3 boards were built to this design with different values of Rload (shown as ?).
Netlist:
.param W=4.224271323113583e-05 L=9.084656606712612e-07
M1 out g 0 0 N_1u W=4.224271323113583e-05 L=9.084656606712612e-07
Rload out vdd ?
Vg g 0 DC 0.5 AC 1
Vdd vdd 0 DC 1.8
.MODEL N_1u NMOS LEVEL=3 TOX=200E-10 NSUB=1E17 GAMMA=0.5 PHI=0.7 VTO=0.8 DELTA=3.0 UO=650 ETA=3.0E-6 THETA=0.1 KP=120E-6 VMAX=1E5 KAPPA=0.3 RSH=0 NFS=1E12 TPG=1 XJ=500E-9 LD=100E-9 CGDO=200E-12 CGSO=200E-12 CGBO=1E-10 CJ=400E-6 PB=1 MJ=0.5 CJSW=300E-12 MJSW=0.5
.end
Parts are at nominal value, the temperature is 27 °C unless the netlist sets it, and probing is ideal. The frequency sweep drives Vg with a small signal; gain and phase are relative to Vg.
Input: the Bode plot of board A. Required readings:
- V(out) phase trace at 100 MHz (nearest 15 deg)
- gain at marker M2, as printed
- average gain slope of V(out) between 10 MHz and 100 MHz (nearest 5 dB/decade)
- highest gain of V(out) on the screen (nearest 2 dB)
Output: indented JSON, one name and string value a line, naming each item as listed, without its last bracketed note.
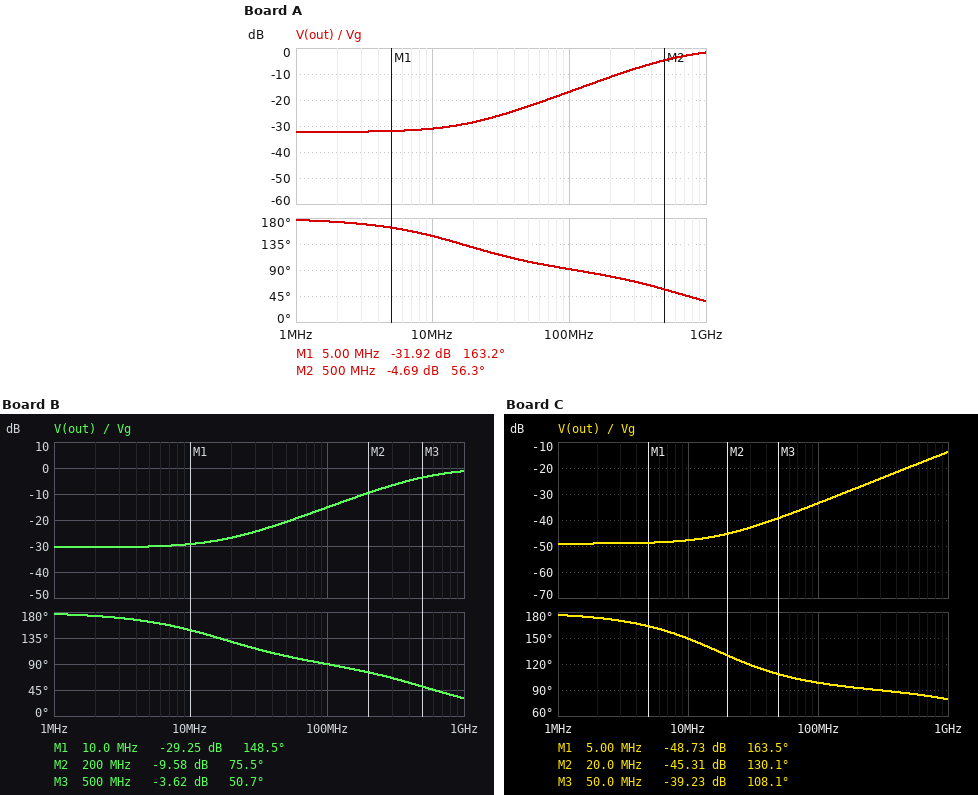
{
  "V(out) phase trace at 100 MHz": "90 deg",
  "gain at marker M2, as printed": "-4.69 dB",
  "average gain slope of V(out) between 10 MHz and 100 MHz": "15 dB/decade",
  "highest gain of V(out) on the screen": "-2 dB"
}
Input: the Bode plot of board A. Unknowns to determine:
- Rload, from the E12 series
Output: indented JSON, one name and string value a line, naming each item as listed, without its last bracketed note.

{
  "Rload, from the E12 series": "27 kΩ"
}
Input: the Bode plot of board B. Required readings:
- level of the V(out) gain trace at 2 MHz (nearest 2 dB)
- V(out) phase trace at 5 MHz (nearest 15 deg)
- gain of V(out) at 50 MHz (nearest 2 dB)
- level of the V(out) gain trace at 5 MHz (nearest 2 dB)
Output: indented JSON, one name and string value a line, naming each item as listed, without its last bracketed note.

{
  "level of the V(out) gain trace at 2 MHz": "-30 dB",
  "V(out) phase trace at 5 MHz": "165 deg",
  "gain of V(out) at 50 MHz": "-20 dB",
  "level of the V(out) gain trace at 5 MHz": "-30 dB"
}
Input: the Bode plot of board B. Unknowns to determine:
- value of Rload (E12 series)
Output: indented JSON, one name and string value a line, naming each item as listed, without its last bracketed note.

{
  "value of Rload": "33 kΩ"
}
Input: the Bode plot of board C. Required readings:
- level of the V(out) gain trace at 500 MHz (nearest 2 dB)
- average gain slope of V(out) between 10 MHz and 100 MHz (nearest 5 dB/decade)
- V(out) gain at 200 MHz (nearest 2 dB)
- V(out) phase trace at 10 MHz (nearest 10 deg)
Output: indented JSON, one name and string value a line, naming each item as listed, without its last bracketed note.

{
  "level of the V(out) gain trace at 500 MHz": "-20 dB",
  "average gain slope of V(out) between 10 MHz and 100 MHz": "15 dB/decade",
  "V(out) gain at 200 MHz": "-28 dB",
  "V(out) phase trace at 10 MHz": "150 deg"
}
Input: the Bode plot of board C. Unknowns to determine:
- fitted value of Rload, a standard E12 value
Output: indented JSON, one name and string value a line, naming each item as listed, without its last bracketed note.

{
  "fitted value of Rload, a standard E12 value": "3.9 kΩ"
}
